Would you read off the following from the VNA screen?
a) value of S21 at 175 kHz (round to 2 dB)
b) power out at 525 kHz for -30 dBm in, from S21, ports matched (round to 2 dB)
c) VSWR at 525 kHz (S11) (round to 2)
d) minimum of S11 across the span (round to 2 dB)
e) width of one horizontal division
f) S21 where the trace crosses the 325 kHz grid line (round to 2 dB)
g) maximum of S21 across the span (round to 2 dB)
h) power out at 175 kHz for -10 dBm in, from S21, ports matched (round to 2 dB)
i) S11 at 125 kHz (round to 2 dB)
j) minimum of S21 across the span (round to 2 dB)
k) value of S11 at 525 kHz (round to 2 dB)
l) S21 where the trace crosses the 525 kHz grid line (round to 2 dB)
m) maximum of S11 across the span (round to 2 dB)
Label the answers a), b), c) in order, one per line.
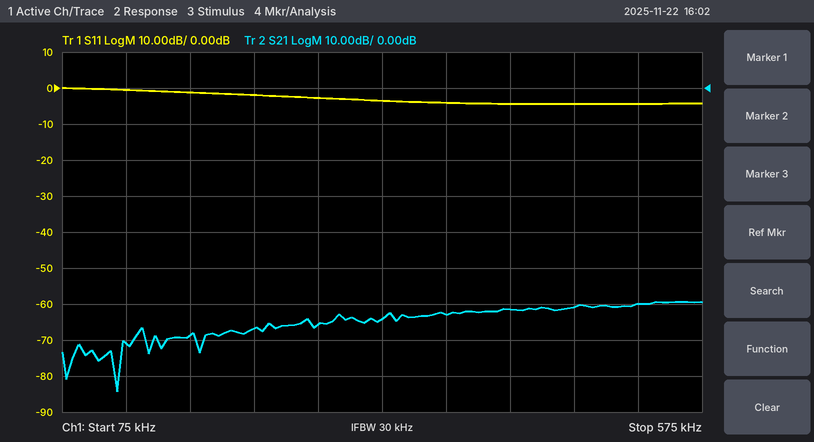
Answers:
a) -68 dB
b) -90 dBm
c) 4
d) -4 dB
e) 50 kHz
f) -64 dB
g) -60 dB
h) -78 dBm
i) 0 dB
j) -84 dB
k) -4 dB
l) -60 dB
m) 0 dB
